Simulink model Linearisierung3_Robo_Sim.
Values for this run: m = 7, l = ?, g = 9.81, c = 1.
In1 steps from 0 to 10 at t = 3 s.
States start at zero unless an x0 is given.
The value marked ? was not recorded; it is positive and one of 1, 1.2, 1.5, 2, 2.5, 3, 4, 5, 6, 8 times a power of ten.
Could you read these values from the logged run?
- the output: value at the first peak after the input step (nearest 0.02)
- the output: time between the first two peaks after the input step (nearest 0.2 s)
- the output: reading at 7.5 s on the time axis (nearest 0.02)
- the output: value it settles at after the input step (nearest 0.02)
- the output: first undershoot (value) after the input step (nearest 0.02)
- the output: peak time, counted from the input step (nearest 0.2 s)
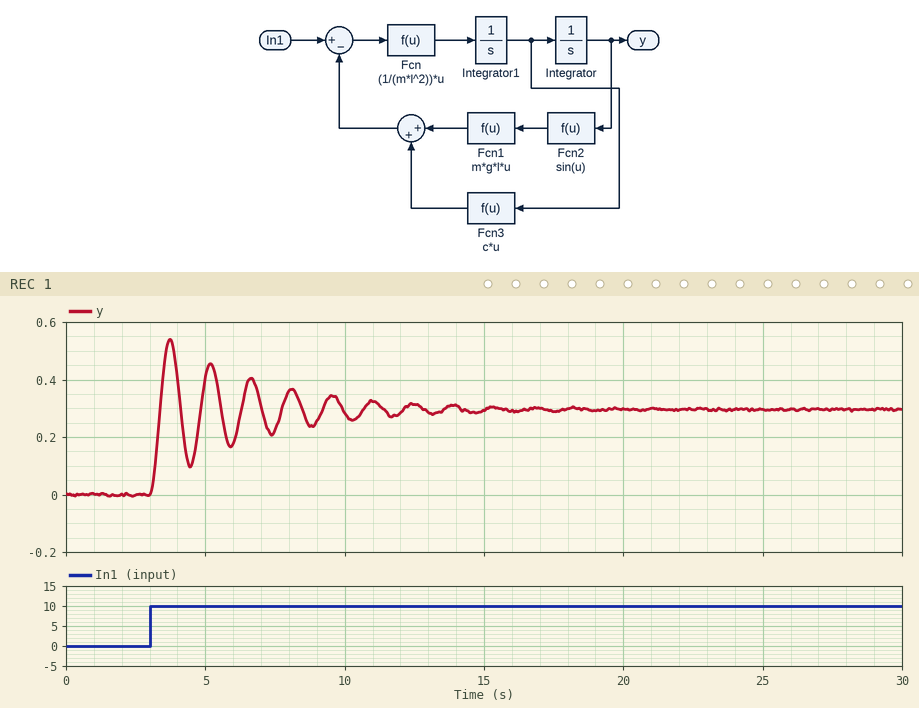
0.54
1.4 s
0.22
0.30
0.10
0.8 s
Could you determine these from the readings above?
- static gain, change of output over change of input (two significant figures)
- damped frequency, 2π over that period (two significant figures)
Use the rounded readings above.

0.030
4.5 rad/s
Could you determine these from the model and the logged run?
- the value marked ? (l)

0.5
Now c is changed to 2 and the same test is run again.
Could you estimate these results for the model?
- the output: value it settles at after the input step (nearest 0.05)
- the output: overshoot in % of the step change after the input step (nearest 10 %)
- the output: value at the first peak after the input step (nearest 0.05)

0.30
70 %
0.50
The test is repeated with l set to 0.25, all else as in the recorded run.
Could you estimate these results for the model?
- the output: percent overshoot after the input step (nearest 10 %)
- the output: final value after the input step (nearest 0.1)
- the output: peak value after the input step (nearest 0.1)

60 %
0.6
1.0
